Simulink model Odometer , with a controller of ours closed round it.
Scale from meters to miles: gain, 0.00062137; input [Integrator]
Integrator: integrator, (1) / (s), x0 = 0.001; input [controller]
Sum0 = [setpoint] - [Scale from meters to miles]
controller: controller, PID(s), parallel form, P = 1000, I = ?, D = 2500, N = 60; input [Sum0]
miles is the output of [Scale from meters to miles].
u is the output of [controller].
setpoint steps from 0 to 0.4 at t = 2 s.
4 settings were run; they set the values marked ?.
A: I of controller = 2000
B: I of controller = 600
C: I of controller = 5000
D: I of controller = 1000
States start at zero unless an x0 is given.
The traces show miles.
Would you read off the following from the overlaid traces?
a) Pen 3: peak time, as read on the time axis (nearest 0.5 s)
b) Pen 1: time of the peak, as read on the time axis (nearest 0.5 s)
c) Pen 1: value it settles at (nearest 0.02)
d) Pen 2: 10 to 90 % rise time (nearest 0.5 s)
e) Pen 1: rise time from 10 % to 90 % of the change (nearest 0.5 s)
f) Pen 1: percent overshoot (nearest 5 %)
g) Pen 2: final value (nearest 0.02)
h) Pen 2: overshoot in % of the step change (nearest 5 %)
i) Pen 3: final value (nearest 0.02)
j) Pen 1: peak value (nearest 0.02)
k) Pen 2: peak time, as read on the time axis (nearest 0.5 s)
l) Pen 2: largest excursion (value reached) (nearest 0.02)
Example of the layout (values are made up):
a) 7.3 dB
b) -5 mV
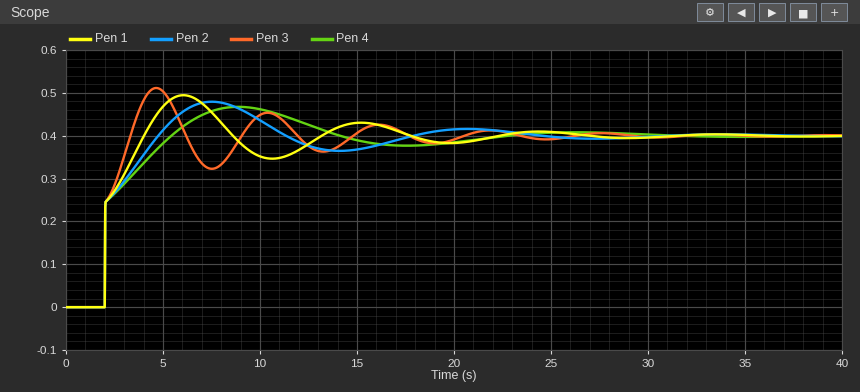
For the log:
a) 4.5 s
b) 6.0 s
c) 0.40
d) 2.0 s
e) 1.5 s
f) 25 %
g) 0.40
h) 20 %
i) 0.40
j) 0.50
k) 7.5 s
l) 0.48
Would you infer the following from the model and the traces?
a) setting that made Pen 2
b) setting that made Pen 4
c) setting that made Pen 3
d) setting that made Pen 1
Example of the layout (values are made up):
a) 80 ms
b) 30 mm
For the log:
a) D
b) B
c) C
d) A
